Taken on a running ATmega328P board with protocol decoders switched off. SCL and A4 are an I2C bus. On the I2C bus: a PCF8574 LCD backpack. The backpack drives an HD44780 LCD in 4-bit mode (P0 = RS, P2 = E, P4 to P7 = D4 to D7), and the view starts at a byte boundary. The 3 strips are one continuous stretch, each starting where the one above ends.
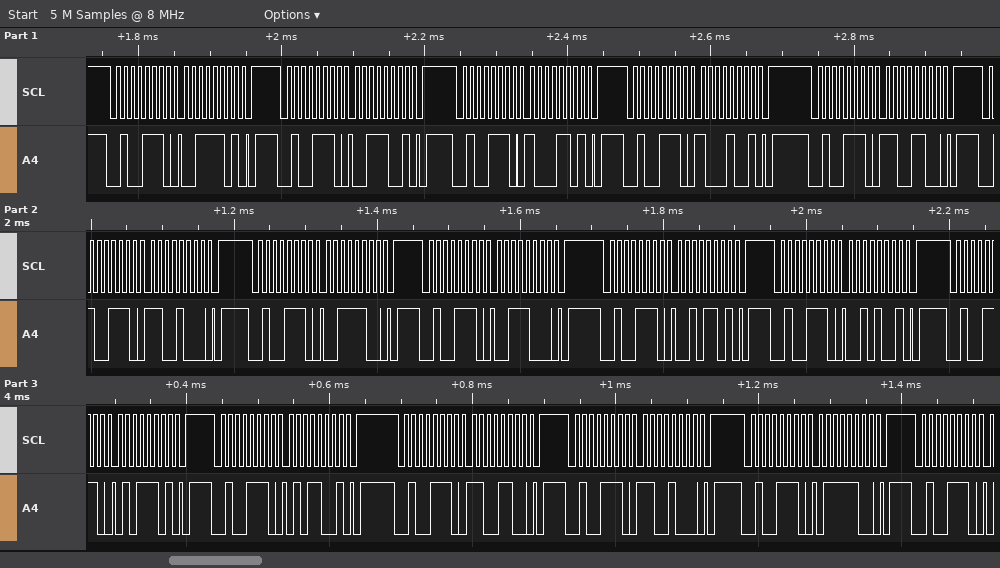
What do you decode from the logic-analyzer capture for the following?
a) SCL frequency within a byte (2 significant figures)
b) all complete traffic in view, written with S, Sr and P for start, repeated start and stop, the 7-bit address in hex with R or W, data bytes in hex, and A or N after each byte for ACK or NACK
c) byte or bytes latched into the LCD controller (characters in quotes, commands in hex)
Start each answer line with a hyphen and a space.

- 100 kHz
- S 27W A 3D A P S 27W A 39 A P S 27W A 8D A P S 27W A 89 A P S 27W A CC A P S 27W A C8 A P S 27W A 3C A P S 27W A 38 A P S 27W A 2D A P S 27W A 29 A P S 27W A 5D A P S 27W A 59 A P S 27W A CC A P S 27W A C8 A P S 27W A 7C A P S 27W A
- '8' 0xC3 '%'
